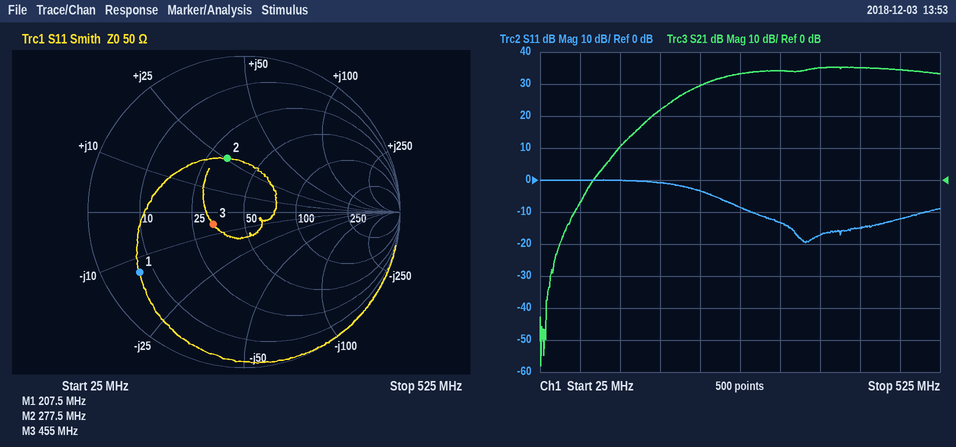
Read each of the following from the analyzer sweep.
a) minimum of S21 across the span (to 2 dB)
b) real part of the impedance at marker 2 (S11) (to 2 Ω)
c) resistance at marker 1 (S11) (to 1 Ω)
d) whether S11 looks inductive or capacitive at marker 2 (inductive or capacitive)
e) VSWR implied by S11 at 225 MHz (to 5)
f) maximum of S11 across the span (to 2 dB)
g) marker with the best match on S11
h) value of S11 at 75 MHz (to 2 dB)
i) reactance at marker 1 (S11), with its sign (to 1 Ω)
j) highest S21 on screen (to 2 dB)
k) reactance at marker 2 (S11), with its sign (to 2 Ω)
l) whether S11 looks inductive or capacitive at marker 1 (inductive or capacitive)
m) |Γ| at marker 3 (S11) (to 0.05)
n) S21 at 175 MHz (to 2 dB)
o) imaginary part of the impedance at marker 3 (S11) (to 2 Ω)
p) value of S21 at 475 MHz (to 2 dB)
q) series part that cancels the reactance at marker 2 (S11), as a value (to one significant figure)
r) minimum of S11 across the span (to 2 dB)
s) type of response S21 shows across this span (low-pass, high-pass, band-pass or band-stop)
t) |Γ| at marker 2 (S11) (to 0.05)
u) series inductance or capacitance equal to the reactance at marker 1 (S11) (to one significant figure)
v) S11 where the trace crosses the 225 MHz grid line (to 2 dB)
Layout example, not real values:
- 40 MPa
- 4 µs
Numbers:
- -58 dB
- 32 Ω
- 7 Ω
- inductive
- 5
- 0 dB
- marker 3
- 0 dB
- -13 Ω
- 36 dB
- +26 Ω
- capacitive
- 0.20
- 22 dB
- -6 Ω
- 34 dB
- 20 pF
- -20 dB
- high-pass
- 0.35
- 60 pF
- -4 dB
